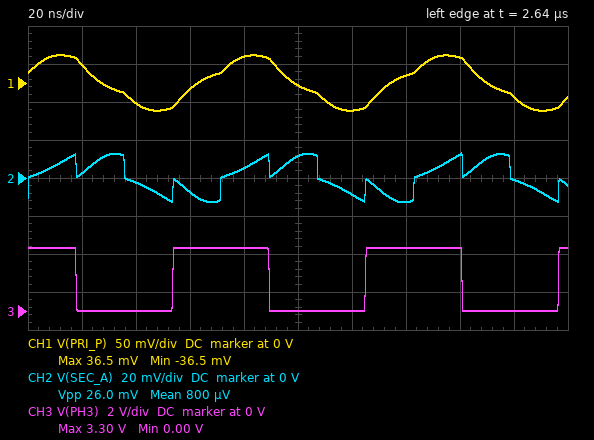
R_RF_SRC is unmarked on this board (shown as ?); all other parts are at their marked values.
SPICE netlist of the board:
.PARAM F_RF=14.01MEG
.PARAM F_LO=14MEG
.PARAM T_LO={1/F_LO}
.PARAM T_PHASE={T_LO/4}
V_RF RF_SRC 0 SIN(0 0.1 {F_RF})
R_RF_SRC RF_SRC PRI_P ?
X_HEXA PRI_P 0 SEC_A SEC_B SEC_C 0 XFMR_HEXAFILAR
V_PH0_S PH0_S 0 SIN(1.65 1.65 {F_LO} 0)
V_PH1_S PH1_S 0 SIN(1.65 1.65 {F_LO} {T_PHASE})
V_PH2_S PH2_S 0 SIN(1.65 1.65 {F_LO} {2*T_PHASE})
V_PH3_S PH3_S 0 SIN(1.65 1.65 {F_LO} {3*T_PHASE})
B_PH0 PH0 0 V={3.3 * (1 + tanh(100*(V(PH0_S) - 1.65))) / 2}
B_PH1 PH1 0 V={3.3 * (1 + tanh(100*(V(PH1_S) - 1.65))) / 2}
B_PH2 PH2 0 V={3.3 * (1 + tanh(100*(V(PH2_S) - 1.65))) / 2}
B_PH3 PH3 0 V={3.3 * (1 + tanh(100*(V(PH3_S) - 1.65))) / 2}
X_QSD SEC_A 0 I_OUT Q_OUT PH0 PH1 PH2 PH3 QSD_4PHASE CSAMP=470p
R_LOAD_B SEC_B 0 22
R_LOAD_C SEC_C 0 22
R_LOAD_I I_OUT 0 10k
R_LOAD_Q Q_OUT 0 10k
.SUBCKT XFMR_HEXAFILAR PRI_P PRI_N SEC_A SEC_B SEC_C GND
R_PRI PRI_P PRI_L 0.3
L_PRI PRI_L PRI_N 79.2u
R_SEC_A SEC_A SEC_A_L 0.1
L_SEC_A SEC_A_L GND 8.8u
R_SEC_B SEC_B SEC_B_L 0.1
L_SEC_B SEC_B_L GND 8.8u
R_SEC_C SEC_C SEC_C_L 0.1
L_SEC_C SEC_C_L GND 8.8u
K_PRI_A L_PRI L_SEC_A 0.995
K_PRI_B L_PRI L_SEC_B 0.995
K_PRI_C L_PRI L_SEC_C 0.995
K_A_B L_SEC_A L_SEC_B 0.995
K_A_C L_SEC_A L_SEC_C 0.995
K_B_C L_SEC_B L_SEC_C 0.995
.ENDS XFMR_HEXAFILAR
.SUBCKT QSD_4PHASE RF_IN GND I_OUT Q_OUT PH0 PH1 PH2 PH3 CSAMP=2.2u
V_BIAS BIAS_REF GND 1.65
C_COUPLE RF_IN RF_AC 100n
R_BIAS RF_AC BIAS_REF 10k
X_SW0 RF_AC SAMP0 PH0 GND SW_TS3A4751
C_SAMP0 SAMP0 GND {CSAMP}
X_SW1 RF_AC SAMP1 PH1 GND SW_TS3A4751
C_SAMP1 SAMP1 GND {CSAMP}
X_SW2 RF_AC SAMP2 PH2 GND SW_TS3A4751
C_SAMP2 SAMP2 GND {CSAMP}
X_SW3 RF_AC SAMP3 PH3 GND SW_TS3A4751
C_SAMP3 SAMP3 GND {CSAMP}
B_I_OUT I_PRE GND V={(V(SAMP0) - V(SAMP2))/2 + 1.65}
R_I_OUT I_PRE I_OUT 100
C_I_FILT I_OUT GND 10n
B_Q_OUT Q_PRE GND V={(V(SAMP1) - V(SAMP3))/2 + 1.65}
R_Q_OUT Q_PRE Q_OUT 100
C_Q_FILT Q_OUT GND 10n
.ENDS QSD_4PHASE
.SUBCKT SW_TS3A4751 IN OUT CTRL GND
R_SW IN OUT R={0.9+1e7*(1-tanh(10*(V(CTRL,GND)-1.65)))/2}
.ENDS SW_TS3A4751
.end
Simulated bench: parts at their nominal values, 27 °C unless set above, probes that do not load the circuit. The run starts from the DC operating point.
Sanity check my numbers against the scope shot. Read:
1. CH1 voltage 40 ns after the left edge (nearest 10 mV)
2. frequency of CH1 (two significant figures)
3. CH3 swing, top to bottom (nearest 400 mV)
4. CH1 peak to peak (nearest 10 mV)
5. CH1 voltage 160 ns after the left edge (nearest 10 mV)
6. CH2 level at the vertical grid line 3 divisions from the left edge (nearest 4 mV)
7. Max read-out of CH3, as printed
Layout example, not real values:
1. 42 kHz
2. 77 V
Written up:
1. -30 mV
2. 14 MHz
3. 3.2 V
4. 70 mV
5. 30 mV
6. -8 mV
7. 3.30 V
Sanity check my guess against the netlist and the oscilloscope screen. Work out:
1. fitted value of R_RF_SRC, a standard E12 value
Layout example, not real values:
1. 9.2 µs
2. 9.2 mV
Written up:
1. 120 Ω
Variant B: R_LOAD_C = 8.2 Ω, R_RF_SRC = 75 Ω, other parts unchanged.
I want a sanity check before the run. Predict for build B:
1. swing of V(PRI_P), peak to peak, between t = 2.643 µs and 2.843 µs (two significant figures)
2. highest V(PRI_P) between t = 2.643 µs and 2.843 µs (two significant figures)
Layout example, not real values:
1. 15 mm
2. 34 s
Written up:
1. 94 mV
2. 47 mV
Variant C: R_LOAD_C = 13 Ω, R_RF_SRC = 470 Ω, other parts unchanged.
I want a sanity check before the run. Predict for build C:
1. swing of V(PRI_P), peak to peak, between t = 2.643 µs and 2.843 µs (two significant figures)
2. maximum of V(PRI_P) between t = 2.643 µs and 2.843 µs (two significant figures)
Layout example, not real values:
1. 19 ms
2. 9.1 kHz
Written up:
1. 23 mV
2. 11 mV
